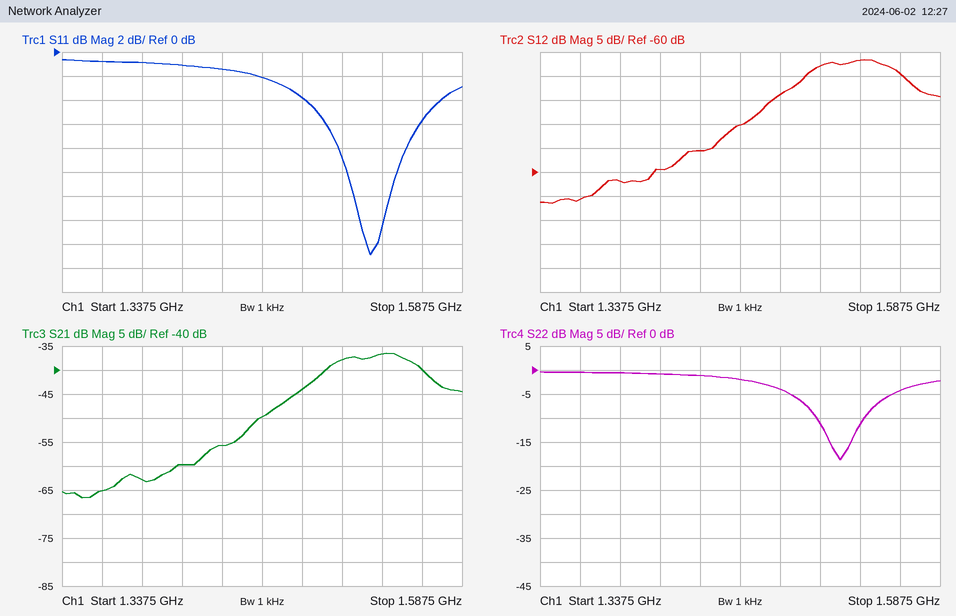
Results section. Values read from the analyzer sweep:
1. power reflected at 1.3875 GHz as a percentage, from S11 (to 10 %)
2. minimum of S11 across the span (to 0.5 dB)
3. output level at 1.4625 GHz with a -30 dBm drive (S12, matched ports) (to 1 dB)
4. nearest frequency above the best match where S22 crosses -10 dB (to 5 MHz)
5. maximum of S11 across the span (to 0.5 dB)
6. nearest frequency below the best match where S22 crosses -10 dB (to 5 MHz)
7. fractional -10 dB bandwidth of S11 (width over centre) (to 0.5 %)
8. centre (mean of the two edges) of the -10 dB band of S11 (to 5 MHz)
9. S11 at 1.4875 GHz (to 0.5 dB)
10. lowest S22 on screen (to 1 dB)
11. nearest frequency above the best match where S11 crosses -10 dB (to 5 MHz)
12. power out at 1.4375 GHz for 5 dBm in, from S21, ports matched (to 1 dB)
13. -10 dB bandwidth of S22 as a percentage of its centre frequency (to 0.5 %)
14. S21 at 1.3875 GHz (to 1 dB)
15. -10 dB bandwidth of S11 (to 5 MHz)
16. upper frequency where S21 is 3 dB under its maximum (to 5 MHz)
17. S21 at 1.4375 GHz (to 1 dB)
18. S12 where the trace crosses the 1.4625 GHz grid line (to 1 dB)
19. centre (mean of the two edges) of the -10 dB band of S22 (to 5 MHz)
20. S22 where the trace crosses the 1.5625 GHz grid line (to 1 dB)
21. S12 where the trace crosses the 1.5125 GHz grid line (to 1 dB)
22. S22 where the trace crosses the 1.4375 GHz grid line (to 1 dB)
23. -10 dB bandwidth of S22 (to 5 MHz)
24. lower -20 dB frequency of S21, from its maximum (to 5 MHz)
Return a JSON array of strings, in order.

["80 %", "-17.0 dB", "-80 dBm", "1.540 GHz", "-0.5 dB", "1.510 GHz", "2.0 %", "1.530 GHz", "-4.0 dB", "-19 dB", "1.545 GHz", "-51 dBm", "2.0 %", "-63 dB", "30 MHz", "1.560 GHz", "-56 dB", "-50 dB", "1.525 GHz", "-4 dB", "-38 dB", "-1 dB", "30 MHz", "1.430 GHz"]
